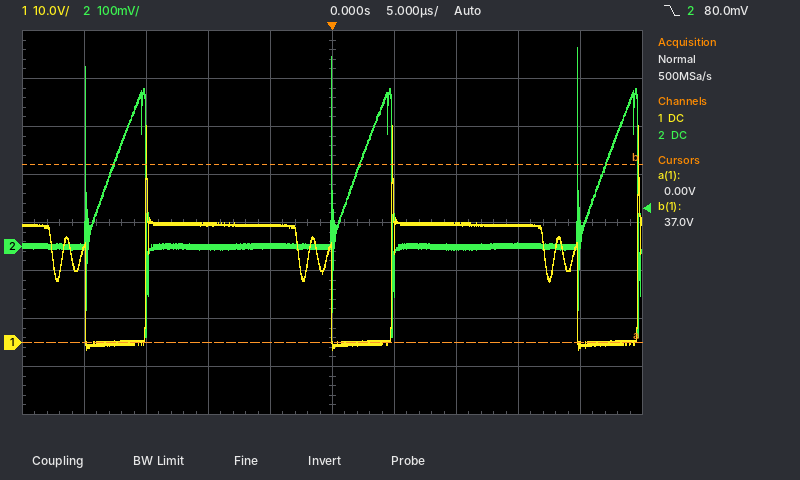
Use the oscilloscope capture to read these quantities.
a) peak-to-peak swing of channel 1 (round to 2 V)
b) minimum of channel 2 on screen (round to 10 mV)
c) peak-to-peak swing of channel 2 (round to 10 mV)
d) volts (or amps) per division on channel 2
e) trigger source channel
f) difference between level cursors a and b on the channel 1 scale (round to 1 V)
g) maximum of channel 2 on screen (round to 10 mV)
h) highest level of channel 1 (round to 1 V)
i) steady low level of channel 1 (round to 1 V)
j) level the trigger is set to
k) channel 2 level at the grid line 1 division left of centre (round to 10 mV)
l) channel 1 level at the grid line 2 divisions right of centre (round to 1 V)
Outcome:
46 V
-190 mV
600 mV
100 mV
channel 2
37 V
410 mV
45 V
0 V
80.0 mV
0 mV
25 V
